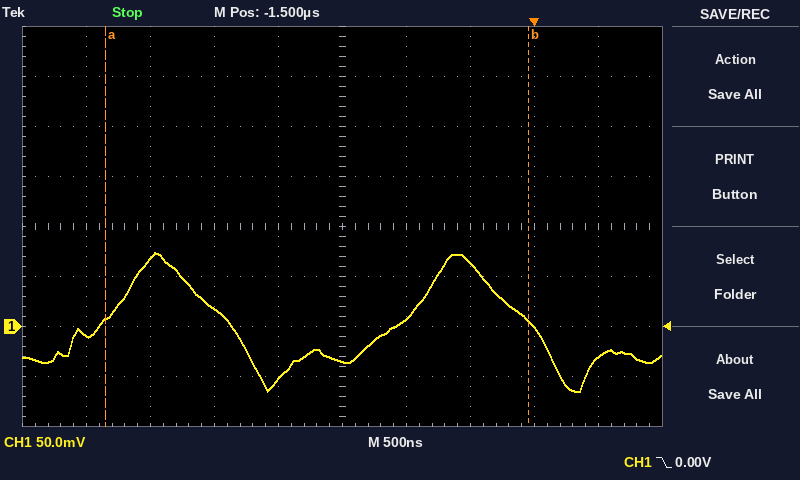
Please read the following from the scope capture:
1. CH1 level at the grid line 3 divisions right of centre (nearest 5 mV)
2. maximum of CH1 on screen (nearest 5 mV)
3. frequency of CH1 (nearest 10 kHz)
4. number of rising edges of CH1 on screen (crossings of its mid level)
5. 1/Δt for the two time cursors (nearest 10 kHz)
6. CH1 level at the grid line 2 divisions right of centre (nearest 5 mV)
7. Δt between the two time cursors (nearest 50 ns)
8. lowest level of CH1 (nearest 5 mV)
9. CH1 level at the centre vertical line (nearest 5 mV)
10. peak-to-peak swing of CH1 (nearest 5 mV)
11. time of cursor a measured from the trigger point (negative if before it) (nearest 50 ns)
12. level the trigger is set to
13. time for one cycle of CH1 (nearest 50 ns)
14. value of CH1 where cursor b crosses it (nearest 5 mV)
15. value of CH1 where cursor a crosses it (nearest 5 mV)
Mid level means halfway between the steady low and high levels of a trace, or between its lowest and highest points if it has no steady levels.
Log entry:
0 mV
75 mV
430 kHz
2
300 kHz
65 mV
3.30 µs
-65 mV
-35 mV
140 mV
-3.35 µs
0.00 V
2.35 µs
5 mV
5 mV
